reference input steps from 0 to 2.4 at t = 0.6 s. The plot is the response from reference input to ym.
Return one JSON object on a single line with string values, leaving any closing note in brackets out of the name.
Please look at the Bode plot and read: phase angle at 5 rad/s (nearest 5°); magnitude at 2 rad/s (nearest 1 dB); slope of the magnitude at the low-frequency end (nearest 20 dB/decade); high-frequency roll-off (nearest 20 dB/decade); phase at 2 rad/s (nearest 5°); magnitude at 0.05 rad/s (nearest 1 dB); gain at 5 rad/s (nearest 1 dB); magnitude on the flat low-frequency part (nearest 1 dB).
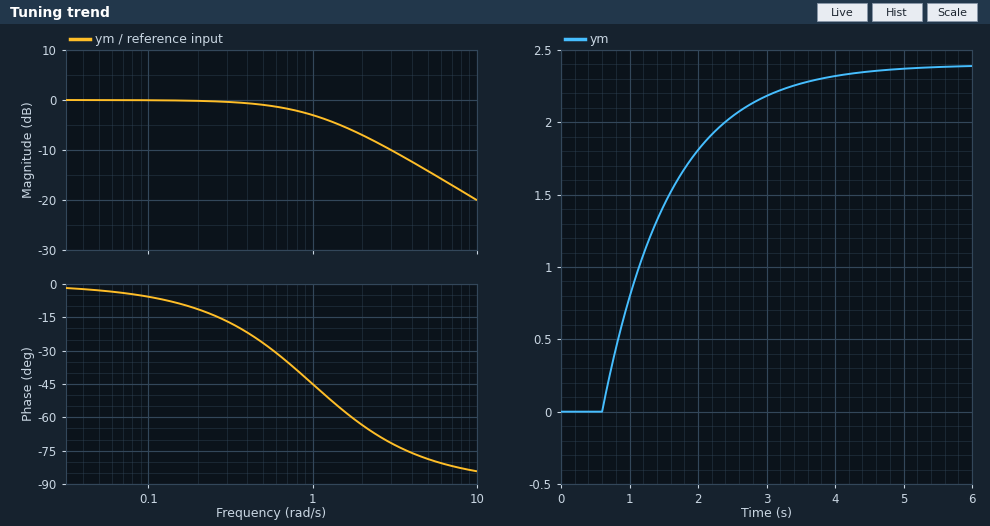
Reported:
{"phase angle at 5 rad/s": "-80°", "magnitude at 2 rad/s": "-7 dB", "slope of the magnitude at the low-frequency end": "0 dB/decade", "high-frequency roll-off": "-20 dB/decade", "phase at 2 rad/s": "-65°", "magnitude at 0.05 rad/s": "0 dB", "gain at 5 rad/s": "-14 dB", "magnitude on the flat low-frequency part": "0 dB"}
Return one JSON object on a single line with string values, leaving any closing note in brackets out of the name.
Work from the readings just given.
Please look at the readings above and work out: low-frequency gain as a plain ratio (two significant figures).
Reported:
{"low-frequency gain as a plain ratio": "1.0"}
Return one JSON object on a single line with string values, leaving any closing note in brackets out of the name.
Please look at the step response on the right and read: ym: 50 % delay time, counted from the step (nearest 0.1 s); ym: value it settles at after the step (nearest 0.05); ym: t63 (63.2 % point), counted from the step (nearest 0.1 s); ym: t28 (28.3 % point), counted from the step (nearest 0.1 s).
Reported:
{"ym: 50 % delay time, counted from the step": "0.7 s", "ym: value it settles at after the step": "2.40", "ym: t63 (63.2 % point), counted from the step": "1.0 s", "ym: t28 (28.3 % point), counted from the step": "0.3 s"}
